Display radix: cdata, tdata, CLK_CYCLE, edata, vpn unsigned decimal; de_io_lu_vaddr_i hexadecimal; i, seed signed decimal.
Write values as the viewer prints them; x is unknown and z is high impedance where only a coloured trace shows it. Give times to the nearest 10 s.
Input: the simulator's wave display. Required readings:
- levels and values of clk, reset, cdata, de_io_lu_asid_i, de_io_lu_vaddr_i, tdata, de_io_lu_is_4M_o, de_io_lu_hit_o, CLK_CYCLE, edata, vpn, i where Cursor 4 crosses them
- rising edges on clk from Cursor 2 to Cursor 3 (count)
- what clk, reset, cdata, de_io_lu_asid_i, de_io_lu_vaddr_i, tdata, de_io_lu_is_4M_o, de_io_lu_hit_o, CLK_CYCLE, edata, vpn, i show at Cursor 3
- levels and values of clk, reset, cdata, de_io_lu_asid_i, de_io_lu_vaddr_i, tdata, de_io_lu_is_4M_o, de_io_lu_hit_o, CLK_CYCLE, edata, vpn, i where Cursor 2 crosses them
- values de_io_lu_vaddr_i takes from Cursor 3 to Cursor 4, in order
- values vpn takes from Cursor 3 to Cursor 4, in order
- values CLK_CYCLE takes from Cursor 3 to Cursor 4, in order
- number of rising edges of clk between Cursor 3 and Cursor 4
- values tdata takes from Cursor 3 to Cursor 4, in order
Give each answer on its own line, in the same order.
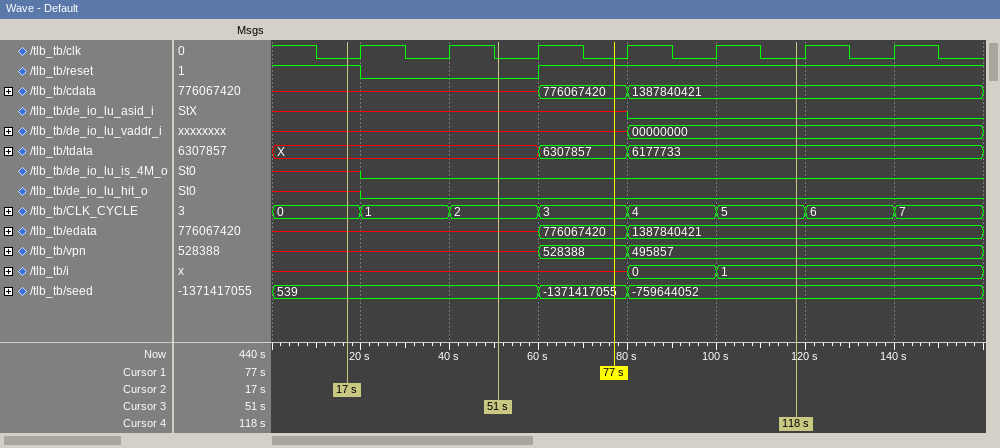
clk=0, reset=1, cdata=1387840421, de_io_lu_asid_i=0, de_io_lu_vaddr_i=00000000, tdata=6177733, de_io_lu_is_4M_o=0, de_io_lu_hit_o=0, CLK_CYCLE=5, edata=1387840421, vpn=495857, i=1
2
clk=0, reset=0, cdata=x, de_io_lu_asid_i=x, de_io_lu_vaddr_i=x, tdata=X, de_io_lu_is_4M_o=0, de_io_lu_hit_o=0, CLK_CYCLE=2, edata=x, vpn=x, i=x
clk=0, reset=1, cdata=x, de_io_lu_asid_i=x, de_io_lu_vaddr_i=x, tdata=X, de_io_lu_is_4M_o=x, de_io_lu_hit_o=x, CLK_CYCLE=0, edata=x, vpn=x, i=x
x, 00000000
x, 528388, 495857
2, 3, 4, 5
3
X, 6307857, 6177733
